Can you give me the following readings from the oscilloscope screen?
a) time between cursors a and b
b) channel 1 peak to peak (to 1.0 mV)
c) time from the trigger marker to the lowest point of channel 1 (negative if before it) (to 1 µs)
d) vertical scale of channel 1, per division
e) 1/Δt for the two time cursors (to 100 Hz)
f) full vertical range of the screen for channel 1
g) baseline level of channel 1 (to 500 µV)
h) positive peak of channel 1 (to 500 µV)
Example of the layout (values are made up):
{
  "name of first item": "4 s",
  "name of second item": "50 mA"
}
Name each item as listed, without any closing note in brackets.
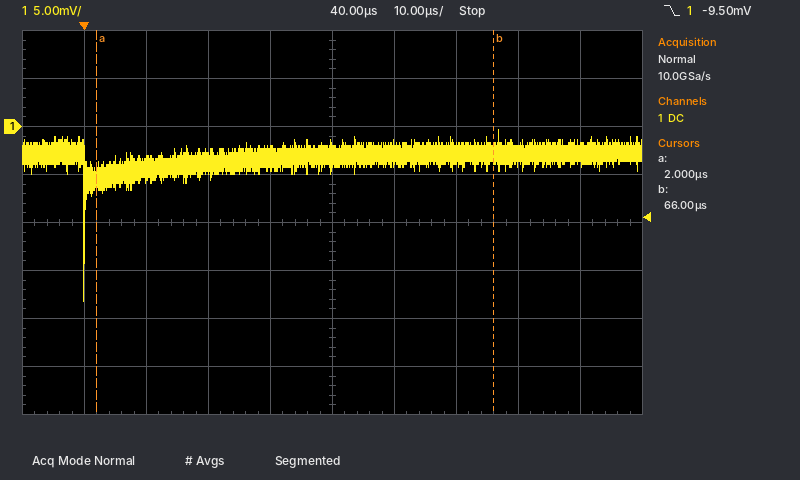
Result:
{
  "time between cursors a and b": "64 µs",
  "channel 1 peak to peak": "18.0 mV",
  "time from the trigger marker to the lowest point of channel 1 (negative if before it)": "0 µs",
  "vertical scale of channel 1, per division": "5 mV",
  "1/Δt for the two time cursors": "15.6 kHz",
  "full vertical range of the screen for channel 1": "40 mV",
  "baseline level of channel 1": "-3.0 mV",
  "positive peak of channel 1": "-500 µV"
}
